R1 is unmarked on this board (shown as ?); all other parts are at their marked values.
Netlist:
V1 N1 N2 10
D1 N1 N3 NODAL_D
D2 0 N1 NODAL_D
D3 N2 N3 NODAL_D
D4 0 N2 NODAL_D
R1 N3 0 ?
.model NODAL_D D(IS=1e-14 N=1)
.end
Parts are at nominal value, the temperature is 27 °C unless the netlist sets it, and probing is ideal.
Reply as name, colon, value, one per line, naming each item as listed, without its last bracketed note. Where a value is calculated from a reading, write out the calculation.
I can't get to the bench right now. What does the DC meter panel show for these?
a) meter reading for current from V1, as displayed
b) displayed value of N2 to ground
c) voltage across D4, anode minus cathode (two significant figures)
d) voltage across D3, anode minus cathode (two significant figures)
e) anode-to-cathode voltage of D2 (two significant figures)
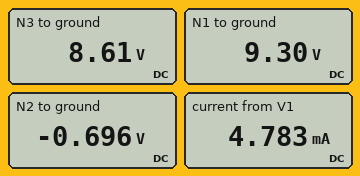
meter reading for current from V1, as displayed: 4.783 mA
displayed value of N2 to ground: -0.696 V
voltage across D4, anode minus cathode: 0 V - (-696 mV) = 700 mV
voltage across D3, anode minus cathode: -696 mV - 8.61 V = -9.3 V
anode-to-cathode voltage of D2: 0 V - 9.3 V = -9.3 V
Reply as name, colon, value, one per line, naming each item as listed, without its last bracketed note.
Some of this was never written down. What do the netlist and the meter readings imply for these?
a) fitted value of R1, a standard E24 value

fitted value of R1, a standard E24 value: 1.8 kΩ
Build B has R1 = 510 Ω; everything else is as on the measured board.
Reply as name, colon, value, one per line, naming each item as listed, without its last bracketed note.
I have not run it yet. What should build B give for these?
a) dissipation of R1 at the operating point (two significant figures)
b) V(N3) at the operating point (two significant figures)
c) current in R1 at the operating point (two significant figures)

dissipation of R1 at the operating point: 140 mW
V(N3) at the operating point: 8.5 V
current in R1 at the operating point: 17 mA
